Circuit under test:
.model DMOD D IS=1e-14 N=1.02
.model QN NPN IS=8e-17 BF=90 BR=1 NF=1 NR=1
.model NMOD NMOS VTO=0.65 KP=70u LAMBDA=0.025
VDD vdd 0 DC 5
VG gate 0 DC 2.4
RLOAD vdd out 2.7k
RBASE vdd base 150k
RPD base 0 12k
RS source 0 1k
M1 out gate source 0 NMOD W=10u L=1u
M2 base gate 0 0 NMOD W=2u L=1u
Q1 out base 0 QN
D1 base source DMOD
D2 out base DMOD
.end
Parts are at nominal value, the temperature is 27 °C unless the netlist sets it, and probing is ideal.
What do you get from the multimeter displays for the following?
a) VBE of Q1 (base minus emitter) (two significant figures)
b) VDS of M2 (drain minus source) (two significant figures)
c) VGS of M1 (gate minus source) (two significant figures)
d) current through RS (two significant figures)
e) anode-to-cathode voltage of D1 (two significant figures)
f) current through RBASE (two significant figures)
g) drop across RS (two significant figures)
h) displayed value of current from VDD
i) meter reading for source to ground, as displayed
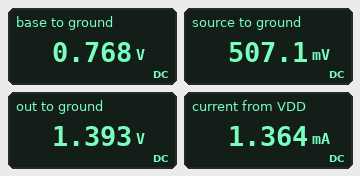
770 mV
770 mV
1.9 V
510 µA
260 mV
28 µA
510 mV
1.364 mA
507.1 mV
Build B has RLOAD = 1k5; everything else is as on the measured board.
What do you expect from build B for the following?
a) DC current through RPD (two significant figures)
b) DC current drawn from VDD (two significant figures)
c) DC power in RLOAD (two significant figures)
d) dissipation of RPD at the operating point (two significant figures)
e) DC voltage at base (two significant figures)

66 µA
2.4 mA
8.5 mW
52 µW
790 mV
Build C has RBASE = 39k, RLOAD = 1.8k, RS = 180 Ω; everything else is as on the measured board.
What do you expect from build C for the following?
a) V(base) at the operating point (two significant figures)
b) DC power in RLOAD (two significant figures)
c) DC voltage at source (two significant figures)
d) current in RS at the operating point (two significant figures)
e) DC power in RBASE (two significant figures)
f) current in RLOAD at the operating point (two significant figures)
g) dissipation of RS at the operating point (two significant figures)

780 mV
7.2 mW
170 mV
950 µA
460 µW
2.0 mA
160 µW
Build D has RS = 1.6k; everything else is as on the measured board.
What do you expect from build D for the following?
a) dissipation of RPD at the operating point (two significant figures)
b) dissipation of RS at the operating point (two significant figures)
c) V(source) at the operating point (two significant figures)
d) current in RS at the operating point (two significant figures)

50 µW
250 µW
640 mV
400 µA
